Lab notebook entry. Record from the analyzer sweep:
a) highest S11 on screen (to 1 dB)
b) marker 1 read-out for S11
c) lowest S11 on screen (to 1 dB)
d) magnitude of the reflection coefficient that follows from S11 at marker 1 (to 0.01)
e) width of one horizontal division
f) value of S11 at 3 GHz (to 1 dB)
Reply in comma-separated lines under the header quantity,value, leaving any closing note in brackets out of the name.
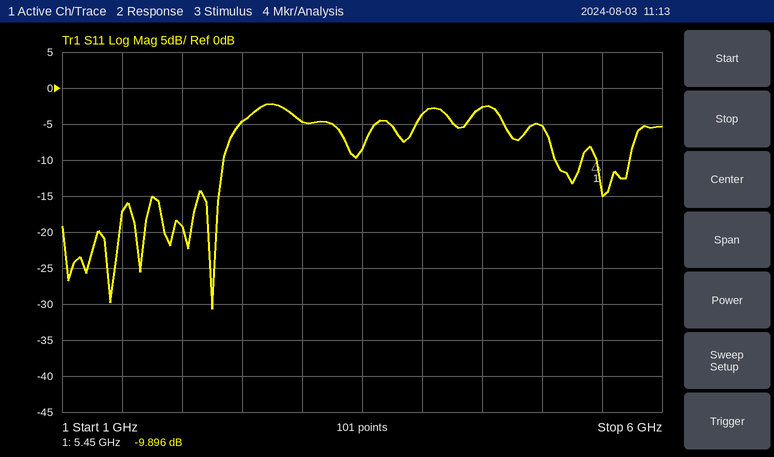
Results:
quantity,value
highest S11 on screen,-2 dB
marker 1 read-out for S11,-9.896 dB
lowest S11 on screen,-31 dB
magnitude of the reflection coefficient that follows from S11 at marker 1,0.32
width of one horizontal division,500 MHz
value of S11 at 3 GHz,-5 dB
